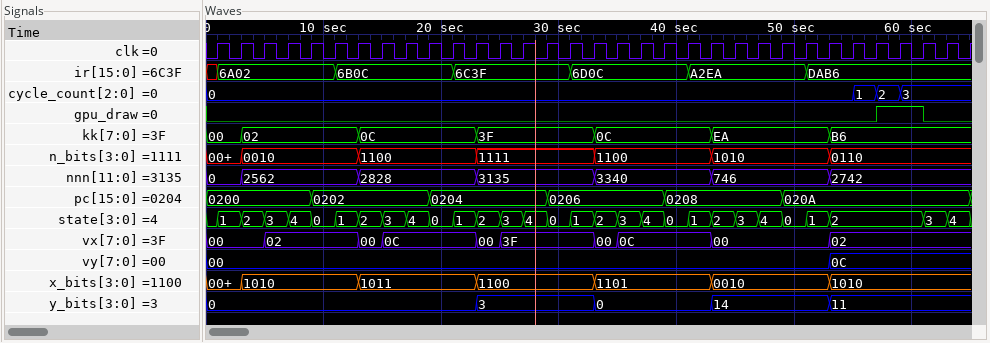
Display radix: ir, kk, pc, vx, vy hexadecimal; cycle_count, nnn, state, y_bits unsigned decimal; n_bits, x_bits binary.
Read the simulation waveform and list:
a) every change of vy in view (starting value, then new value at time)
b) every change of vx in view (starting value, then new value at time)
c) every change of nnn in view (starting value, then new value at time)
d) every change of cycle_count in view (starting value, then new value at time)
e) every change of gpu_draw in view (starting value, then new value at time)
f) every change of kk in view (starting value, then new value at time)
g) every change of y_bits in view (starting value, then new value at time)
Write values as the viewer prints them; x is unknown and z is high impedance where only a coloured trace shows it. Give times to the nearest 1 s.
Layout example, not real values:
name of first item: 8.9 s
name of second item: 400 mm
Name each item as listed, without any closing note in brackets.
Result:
every change of vy in view: 00, 0C at 53 s
every change of vx in view: 00, 02 at 5 s, 00 at 13 s, 0C at 15 s, 00 at 23 s, 3F at 25 s, 00 at 33 s, 0C at 35 s, 00 at 43 s, 02 at 53 s
every change of nnn in view: 0, 2562 at 3 s, 2828 at 13 s, 3135 at 23 s, 3340 at 33 s, 746 at 43 s, 2742 at 53 s
every change of cycle_count in view: 0, 1 at 55 s, 2 at 57 s, 3 at 59 s
every change of gpu_draw in view: 0, 1 at 57 s, 0 at 61 s
every change of kk in view: 00, 02 at 3 s, 0C at 13 s, 3F at 23 s, 0C at 33 s, EA at 43 s, B6 at 53 s
every change of y_bits in view: 0, 3 at 23 s, 0 at 33 s, 14 at 43 s, 11 at 53 s
